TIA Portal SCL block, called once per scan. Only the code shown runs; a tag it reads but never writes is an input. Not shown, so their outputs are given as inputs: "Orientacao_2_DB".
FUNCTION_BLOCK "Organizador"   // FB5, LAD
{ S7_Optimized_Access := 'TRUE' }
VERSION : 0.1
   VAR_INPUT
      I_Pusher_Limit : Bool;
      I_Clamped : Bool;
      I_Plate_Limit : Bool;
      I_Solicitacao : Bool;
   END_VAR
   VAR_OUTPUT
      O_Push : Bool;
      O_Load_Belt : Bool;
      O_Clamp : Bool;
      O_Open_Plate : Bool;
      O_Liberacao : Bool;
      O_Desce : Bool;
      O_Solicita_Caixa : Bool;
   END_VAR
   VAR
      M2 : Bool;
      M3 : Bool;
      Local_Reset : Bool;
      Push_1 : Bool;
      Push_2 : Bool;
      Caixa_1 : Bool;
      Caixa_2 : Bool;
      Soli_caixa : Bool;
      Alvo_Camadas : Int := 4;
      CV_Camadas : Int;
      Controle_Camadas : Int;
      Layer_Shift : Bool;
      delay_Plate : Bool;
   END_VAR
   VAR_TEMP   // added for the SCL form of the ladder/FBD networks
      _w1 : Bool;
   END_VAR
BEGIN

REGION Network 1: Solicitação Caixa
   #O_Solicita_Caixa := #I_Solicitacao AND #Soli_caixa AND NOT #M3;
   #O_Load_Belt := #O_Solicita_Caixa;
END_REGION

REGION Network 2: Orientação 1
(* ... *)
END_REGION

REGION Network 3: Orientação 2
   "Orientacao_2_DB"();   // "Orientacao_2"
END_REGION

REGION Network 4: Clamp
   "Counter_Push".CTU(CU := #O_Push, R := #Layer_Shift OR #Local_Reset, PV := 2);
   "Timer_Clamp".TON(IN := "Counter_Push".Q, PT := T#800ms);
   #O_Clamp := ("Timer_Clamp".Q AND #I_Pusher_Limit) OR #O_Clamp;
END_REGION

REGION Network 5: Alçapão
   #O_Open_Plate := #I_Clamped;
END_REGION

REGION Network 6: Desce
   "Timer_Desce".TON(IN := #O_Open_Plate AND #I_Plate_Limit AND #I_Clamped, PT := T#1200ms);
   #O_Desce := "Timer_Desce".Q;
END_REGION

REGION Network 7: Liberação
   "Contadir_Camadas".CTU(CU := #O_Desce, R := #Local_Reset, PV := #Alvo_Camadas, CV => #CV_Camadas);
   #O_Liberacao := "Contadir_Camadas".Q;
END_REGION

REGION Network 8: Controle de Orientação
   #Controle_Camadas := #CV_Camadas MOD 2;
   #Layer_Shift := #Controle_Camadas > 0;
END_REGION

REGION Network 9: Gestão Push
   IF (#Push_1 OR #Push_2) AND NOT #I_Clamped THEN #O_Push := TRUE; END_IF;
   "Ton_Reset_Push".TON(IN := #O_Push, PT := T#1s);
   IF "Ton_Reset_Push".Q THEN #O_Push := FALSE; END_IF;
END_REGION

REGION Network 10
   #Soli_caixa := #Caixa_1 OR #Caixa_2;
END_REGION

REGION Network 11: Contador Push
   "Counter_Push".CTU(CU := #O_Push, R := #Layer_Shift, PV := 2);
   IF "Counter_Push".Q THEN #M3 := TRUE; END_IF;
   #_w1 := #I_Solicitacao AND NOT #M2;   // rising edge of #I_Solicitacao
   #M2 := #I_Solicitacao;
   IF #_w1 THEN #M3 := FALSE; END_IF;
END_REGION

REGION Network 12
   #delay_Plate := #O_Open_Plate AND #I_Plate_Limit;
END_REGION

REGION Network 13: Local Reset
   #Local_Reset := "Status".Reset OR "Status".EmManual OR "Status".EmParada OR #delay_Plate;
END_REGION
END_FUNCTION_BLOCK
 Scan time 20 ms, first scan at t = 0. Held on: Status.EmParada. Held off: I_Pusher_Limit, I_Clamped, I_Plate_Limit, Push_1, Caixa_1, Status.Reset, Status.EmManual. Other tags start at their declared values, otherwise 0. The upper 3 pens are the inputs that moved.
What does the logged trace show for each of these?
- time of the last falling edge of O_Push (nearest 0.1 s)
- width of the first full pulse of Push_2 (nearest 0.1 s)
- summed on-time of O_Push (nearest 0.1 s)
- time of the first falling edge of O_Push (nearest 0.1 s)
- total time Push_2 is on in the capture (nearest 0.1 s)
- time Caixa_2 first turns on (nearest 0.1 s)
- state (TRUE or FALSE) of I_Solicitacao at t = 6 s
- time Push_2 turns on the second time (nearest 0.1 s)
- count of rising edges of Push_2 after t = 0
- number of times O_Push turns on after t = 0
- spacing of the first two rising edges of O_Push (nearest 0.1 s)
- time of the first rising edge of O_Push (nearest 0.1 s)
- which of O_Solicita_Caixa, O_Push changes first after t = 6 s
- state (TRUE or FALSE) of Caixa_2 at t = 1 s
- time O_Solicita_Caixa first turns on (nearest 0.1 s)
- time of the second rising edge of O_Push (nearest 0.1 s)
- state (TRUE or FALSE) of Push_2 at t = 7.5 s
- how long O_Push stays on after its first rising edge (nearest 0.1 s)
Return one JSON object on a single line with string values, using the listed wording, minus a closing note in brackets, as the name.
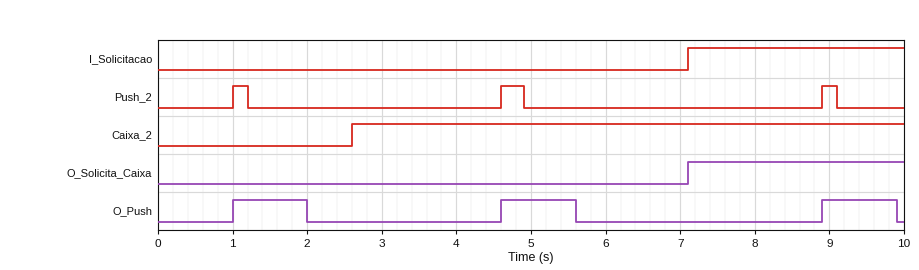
{"time of the last falling edge of O_Push": "9.9 s", "width of the first full pulse of Push_2": "0.2 s", "summed on-time of O_Push": "3.0 s", "time of the first falling edge of O_Push": "2.0 s", "total time Push_2 is on in the capture": "0.7 s", "time Caixa_2 first turns on": "2.6 s", "state (TRUE or FALSE) of I_Solicitacao at t = 6 s": "FALSE", "time Push_2 turns on the second time": "4.6 s", "count of rising edges of Push_2 after t = 0": "3", "number of times O_Push turns on after t = 0": "3", "spacing of the first two rising edges of O_Push": "3.6 s", "time of the first rising edge of O_Push": "1.0 s", "which of O_Solicita_Caixa, O_Push changes first after t = 6 s": "O_Solicita_Caixa", "state (TRUE or FALSE) of Caixa_2 at t = 1 s": "FALSE", "time O_Solicita_Caixa first turns on": "7.1 s", "time of the second rising edge of O_Push": "4.6 s", "state (TRUE or FALSE) of Push_2 at t = 7.5 s": "FALSE", "how long O_Push stays on after its first rising edge": "1.0 s"}
